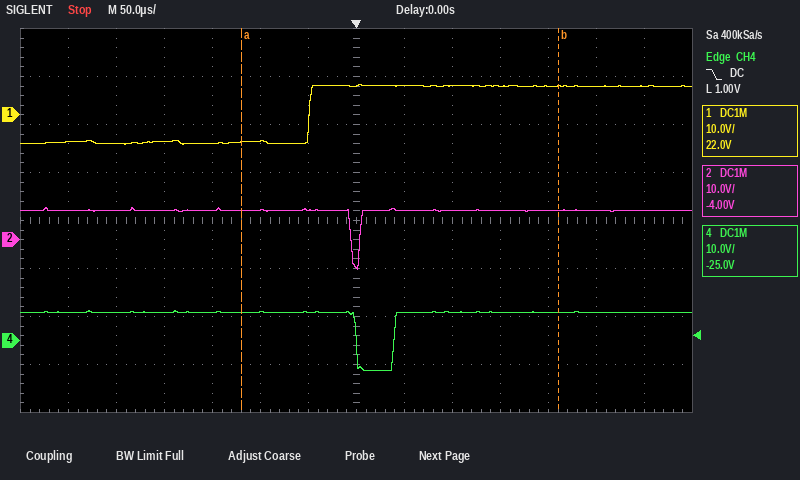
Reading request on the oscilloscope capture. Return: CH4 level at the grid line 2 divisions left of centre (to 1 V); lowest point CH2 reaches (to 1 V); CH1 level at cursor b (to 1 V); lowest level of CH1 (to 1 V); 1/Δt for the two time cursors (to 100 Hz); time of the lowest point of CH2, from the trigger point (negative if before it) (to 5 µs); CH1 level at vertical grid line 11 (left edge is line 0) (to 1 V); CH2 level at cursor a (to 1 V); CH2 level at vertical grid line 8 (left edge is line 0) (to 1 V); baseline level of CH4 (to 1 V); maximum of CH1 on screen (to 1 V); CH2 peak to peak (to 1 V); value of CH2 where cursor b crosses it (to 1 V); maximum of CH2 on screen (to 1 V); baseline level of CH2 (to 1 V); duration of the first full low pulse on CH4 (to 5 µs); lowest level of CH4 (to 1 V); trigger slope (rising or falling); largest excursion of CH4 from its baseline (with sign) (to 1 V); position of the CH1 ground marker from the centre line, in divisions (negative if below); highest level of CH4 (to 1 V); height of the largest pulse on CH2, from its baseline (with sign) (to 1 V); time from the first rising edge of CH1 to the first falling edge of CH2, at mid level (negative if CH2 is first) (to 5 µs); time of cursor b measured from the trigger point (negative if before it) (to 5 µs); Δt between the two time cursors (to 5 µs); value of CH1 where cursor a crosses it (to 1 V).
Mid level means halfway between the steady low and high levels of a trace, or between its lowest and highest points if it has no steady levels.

6 V
-6 V
6 V
-6 V
3.0 kHz
0 µs
6 V
6 V
6 V
6 V
6 V
13 V
6 V
7 V
6 V
40 µs
-6 V
falling
-12 V
+2.2 div
6 V
-12 V
+45 µs
+210 µs
330 µs
-6 V
